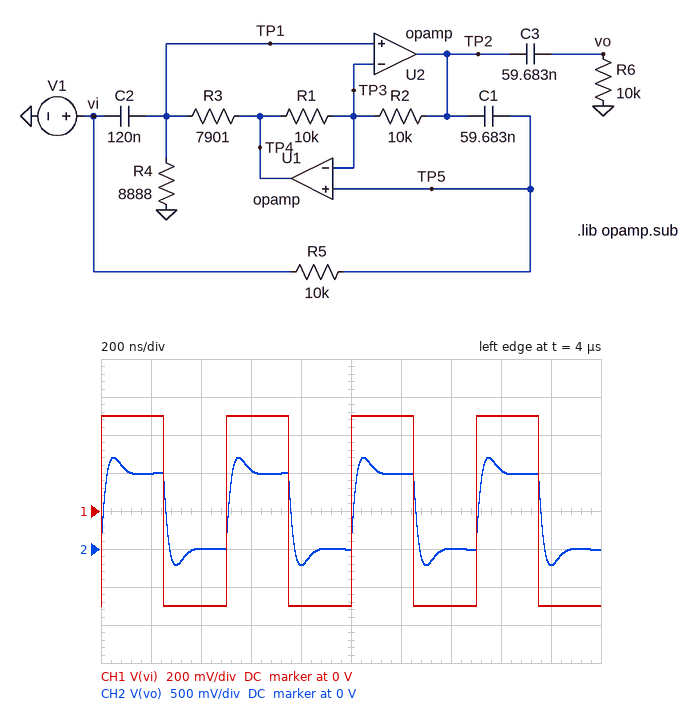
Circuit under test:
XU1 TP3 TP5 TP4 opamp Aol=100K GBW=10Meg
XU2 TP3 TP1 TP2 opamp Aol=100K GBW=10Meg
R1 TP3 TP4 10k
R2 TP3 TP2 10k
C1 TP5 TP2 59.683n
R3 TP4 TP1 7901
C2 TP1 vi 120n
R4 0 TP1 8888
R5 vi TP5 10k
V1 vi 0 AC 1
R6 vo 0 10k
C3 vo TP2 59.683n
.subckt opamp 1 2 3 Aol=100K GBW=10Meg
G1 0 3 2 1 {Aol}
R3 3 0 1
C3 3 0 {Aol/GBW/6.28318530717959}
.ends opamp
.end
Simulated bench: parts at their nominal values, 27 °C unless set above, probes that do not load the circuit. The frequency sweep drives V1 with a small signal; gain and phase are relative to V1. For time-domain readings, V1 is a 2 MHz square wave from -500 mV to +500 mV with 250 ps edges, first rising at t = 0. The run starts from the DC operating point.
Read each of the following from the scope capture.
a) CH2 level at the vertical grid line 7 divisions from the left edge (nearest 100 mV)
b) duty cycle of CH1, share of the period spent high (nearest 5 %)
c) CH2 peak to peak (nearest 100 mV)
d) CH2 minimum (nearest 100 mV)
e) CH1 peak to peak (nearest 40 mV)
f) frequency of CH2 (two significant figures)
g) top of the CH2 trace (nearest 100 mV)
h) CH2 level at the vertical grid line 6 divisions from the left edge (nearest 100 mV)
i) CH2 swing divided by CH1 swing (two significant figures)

0 V
50 %
1.4 V
-200 mV
1.00 V
2.0 MHz
1.2 V
1.0 V
1.4
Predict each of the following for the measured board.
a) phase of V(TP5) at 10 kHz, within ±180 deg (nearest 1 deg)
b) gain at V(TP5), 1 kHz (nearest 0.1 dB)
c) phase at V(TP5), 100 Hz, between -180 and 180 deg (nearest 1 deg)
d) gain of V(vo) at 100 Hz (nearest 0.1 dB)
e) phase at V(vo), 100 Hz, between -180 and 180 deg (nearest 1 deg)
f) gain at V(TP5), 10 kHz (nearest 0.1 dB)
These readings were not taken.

1 deg
-0.1 dB
-23 deg
-26.6 dB
-134 deg
0 dB
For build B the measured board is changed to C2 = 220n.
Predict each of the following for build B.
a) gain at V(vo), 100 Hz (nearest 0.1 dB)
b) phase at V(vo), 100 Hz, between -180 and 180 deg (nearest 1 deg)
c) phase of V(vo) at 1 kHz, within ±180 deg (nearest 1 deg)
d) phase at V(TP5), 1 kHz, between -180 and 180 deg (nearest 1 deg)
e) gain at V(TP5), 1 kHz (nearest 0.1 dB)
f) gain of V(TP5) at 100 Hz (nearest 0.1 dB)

-16.2 dB
-140 deg
20 deg
5 deg
0 dB
-1.2 dB
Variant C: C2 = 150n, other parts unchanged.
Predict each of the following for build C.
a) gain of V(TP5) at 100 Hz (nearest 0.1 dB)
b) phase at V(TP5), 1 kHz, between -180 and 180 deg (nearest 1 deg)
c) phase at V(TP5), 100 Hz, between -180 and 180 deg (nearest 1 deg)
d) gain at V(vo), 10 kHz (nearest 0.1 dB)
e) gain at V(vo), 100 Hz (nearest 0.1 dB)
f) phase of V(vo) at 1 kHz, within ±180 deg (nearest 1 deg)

-0.8 dB
7 deg
-25 deg
0 dB
-22.6 dB
22 deg
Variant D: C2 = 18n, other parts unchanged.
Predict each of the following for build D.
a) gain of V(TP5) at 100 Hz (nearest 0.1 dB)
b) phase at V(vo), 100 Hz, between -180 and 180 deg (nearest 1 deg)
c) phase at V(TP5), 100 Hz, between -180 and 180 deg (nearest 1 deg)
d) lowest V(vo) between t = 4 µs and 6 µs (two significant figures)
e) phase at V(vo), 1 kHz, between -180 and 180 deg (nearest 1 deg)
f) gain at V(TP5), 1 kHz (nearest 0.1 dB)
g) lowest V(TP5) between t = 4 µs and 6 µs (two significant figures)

-0.5 dB
50 deg
-19 deg
-230 mV
70 deg
-4.8 dB
-730 mV
